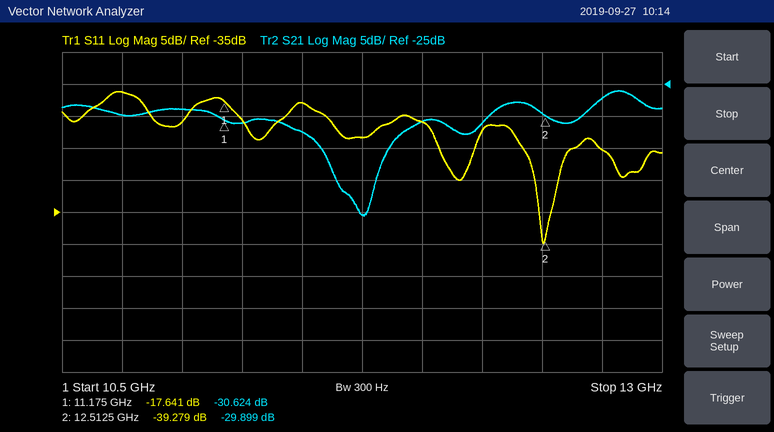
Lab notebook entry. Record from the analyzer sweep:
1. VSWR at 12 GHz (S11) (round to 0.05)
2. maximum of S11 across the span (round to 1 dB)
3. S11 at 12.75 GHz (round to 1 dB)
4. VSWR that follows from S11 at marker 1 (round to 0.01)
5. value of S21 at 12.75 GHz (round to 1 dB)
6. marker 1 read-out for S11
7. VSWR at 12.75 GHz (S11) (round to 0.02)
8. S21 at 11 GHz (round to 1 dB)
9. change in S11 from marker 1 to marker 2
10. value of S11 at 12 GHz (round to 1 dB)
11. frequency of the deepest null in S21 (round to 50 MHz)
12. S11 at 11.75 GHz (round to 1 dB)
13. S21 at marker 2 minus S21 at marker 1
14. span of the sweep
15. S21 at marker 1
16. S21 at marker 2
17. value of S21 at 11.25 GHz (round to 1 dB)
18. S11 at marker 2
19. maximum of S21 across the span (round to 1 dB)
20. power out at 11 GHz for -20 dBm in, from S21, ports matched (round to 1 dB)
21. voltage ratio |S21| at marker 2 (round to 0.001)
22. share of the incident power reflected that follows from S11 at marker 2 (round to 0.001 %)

1.20
-16 dB
-25 dB
1.30
-27 dB
-17.641 dB
1.12
-29 dB
-21.638 dB
-21 dB
11.75 GHz
-23 dB
0.725 dB
2.5 GHz
-30.624 dB
-29.899 dB
-31 dB
-39.279 dB
-26 dB
-49 dBm
0.032
0.012 %
